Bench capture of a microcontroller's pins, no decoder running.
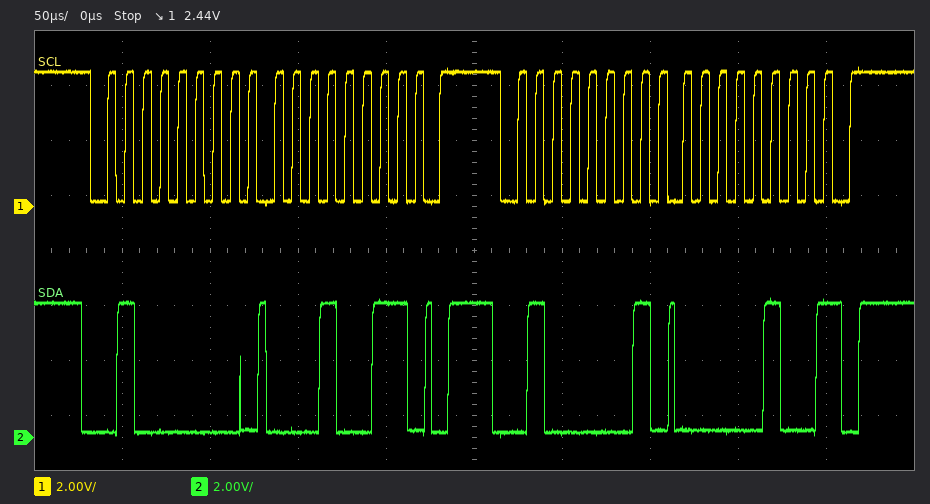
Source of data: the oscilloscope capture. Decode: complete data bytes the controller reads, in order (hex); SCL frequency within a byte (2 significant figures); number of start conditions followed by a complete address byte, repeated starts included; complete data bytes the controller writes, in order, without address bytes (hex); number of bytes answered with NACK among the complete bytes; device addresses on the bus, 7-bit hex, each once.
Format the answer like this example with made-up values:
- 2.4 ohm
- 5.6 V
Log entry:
- 04
- 100 kHz
- 2
- 13
- 1
- 0x20
